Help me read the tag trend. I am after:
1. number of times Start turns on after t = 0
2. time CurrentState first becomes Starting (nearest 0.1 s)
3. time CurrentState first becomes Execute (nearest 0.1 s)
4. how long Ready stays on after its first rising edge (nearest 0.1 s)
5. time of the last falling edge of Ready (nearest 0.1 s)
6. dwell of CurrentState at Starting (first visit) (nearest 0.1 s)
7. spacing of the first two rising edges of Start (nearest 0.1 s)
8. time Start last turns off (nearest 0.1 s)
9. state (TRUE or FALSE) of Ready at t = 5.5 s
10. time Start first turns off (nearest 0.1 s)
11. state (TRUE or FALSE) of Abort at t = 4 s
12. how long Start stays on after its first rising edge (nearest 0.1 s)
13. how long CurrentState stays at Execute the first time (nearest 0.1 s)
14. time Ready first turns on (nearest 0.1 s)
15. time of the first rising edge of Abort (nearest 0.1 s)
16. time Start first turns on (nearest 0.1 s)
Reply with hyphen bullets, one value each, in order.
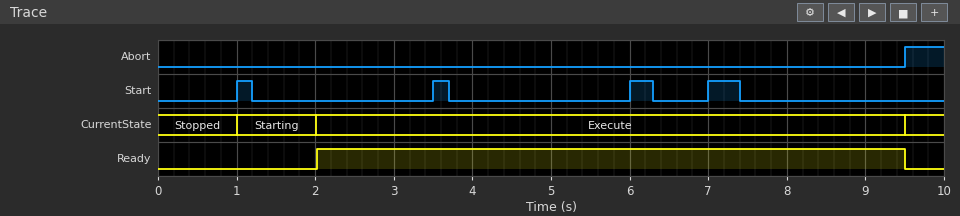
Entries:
- 4
- 1.0 s
- 2.0 s
- 7.5 s
- 9.5 s
- 1.0 s
- 2.5 s
- 7.4 s
- TRUE
- 1.2 s
- FALSE
- 0.2 s
- 7.5 s
- 2.0 s
- 9.5 s
- 1.0 s
